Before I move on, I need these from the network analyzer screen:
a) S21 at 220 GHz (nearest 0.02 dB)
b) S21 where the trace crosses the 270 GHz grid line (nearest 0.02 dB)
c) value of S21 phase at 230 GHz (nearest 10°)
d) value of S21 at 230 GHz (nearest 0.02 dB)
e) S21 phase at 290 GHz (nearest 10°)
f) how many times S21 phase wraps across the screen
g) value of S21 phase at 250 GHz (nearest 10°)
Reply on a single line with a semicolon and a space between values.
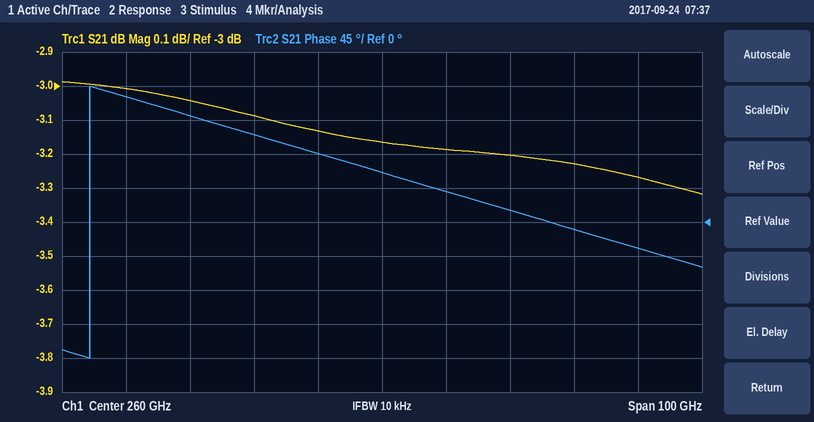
-3.00 dB; -3.18 dB; 140°; -3.04 dB; -10°; 1; 90°
